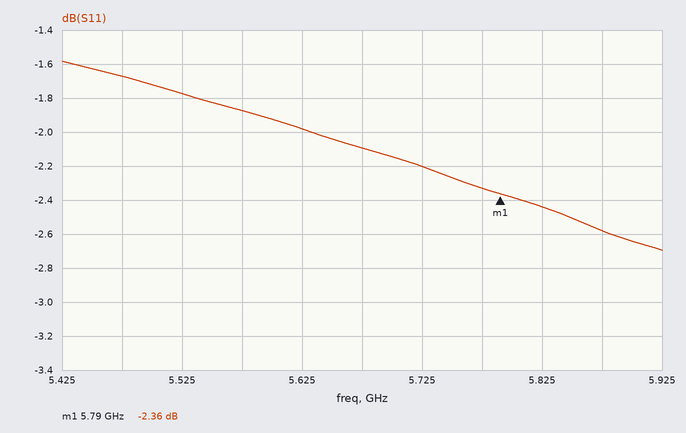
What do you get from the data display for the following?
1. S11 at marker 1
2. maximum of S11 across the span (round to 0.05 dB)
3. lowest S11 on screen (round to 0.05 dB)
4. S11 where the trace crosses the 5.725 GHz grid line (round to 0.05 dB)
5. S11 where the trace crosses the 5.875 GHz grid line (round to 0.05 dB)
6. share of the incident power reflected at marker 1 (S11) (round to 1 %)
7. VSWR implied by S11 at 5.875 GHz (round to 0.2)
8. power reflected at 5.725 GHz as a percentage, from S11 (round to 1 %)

-2.36 dB
-1.60 dB
-2.70 dB
-2.20 dB
-2.60 dB
58 %
6.8
60 %
